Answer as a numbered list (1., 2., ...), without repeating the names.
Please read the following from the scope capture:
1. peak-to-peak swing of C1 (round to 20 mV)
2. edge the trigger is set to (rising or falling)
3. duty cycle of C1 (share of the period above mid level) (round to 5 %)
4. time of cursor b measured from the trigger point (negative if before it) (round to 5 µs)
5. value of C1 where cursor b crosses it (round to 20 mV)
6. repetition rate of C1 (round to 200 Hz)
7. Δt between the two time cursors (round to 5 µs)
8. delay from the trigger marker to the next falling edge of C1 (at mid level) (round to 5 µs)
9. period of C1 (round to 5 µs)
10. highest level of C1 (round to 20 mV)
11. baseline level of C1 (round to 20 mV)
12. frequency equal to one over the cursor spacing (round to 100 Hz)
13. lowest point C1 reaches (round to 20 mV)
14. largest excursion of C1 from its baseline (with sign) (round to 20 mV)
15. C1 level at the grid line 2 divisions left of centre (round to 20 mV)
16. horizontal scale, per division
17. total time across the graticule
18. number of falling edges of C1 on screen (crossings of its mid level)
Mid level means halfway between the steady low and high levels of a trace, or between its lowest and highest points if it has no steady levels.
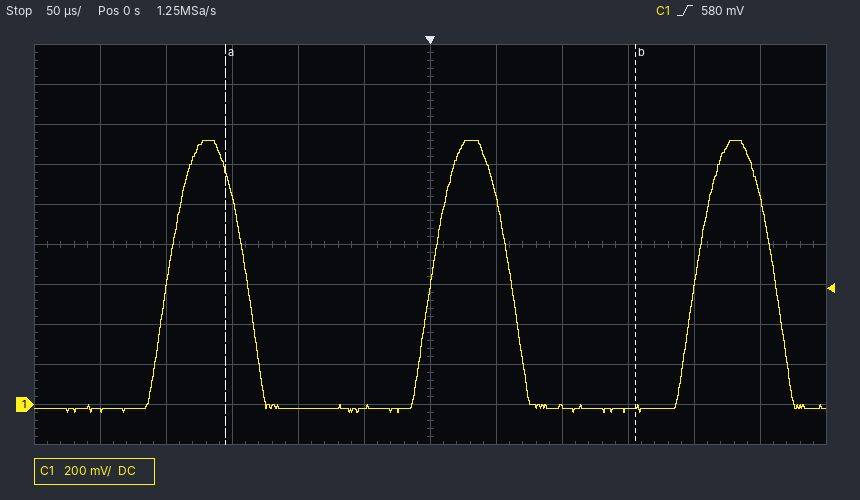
1. 1.36 V
2. rising
3. 30 %
4. +155 µs
5. -20 mV
6. 5.0 kHz
7. 310 µs
8. 60 µs
9. 200 µs
10. 1.32 V
11. -20 mV
12. 3.2 kHz
13. -40 mV
14. +1.34 V
15. -20 mV
16. 50 µs
17. 600 µs
18. 3
